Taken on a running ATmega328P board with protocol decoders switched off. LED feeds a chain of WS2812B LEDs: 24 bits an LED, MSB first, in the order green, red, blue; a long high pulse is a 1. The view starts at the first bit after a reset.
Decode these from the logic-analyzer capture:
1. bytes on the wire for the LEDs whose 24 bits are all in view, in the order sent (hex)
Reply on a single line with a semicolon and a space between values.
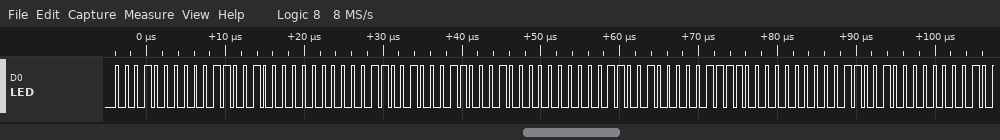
10 32 00 32 31 00 32 0F 00
